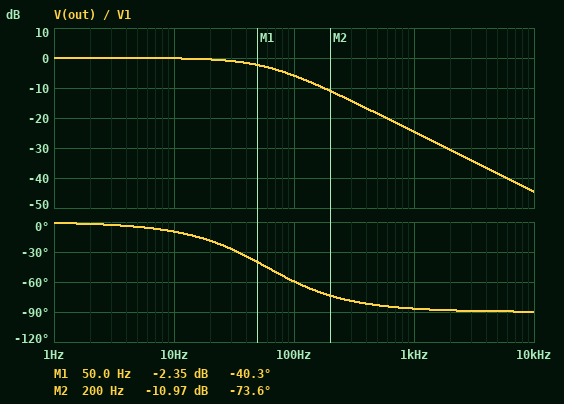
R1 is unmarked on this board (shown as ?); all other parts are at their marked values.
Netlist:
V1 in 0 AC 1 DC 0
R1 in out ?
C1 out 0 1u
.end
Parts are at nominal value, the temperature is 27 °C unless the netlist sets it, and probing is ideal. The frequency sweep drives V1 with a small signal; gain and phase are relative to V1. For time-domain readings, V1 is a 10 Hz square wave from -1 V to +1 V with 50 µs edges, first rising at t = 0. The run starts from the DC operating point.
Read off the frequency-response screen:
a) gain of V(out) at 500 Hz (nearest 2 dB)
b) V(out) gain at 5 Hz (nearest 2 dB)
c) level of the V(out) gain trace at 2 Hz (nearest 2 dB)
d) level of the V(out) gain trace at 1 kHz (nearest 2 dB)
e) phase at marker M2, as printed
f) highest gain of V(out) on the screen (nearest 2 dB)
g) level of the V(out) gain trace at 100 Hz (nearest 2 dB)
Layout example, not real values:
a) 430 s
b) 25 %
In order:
a) -18 dB
b) 0 dB
c) 0 dB
d) -24 dB
e) -73.6 deg
f) 0 dB
g) -6 dB
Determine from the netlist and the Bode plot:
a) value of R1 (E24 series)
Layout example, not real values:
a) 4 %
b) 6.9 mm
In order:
a) 2.7 kΩ
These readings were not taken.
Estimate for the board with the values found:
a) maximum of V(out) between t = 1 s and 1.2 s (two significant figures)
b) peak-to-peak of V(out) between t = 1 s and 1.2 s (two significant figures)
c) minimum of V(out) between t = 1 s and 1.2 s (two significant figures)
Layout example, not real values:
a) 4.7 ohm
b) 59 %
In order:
a) 1.0 V
b) 2.0 V
c) -1.0 V
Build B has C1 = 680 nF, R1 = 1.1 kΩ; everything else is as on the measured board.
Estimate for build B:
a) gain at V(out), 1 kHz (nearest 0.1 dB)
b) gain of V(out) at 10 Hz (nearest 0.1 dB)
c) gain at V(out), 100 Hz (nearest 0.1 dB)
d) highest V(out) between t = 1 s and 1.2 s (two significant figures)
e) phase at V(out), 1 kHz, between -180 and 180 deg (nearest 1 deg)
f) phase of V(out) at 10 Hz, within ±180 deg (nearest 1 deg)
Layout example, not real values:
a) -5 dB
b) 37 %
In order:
a) -13.6 dB
b) 0 dB
c) -0.9 dB
d) 1.0 V
e) -78 deg
f) -3 deg
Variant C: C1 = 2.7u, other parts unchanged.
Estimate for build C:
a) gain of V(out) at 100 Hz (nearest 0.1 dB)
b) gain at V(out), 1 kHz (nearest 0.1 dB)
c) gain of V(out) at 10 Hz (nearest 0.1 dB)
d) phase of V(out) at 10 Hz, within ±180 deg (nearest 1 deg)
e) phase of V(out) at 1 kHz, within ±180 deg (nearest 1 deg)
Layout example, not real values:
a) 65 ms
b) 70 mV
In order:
a) -13.4 dB
b) -33.2 dB
c) -0.8 dB
d) -25 deg
e) -89 deg
